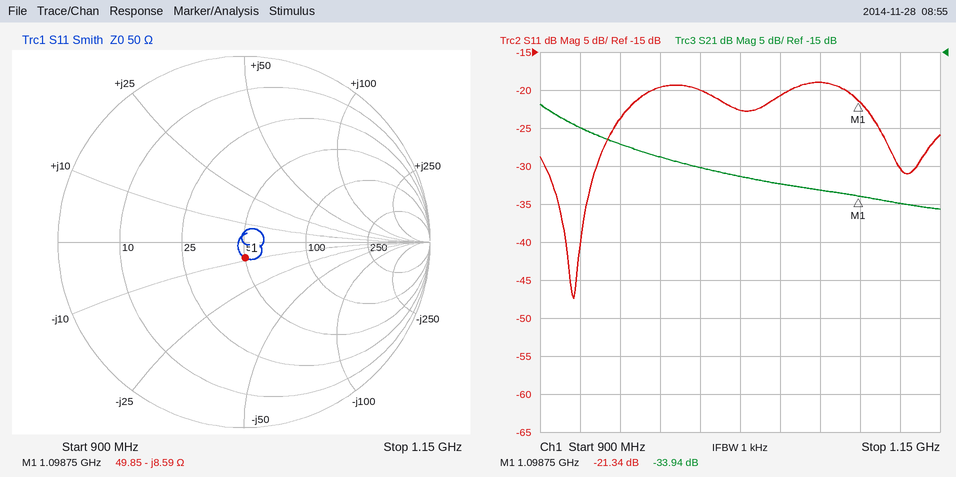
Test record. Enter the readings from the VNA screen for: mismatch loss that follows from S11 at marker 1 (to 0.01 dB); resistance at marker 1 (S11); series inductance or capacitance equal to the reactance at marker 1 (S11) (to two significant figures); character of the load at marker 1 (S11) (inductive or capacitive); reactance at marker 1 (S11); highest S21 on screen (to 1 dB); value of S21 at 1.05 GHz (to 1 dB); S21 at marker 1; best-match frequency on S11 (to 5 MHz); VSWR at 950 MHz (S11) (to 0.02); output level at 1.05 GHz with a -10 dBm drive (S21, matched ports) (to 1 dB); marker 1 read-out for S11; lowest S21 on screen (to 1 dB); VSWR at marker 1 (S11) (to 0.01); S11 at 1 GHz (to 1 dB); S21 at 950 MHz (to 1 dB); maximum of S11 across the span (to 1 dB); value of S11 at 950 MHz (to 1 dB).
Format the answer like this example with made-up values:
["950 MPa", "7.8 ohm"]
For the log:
["0.03 dB", "49.85 Ω", "17 pF", "capacitive", "-8.59 Ω", "-22 dB", "-32 dB", "-33.94 dB", "920 MHz", "1.14", "-42 dBm", "-21.34 dB", "-36 dB", "1.19", "-20 dB", "-27 dB", "-19 dB", "-24 dB"]
